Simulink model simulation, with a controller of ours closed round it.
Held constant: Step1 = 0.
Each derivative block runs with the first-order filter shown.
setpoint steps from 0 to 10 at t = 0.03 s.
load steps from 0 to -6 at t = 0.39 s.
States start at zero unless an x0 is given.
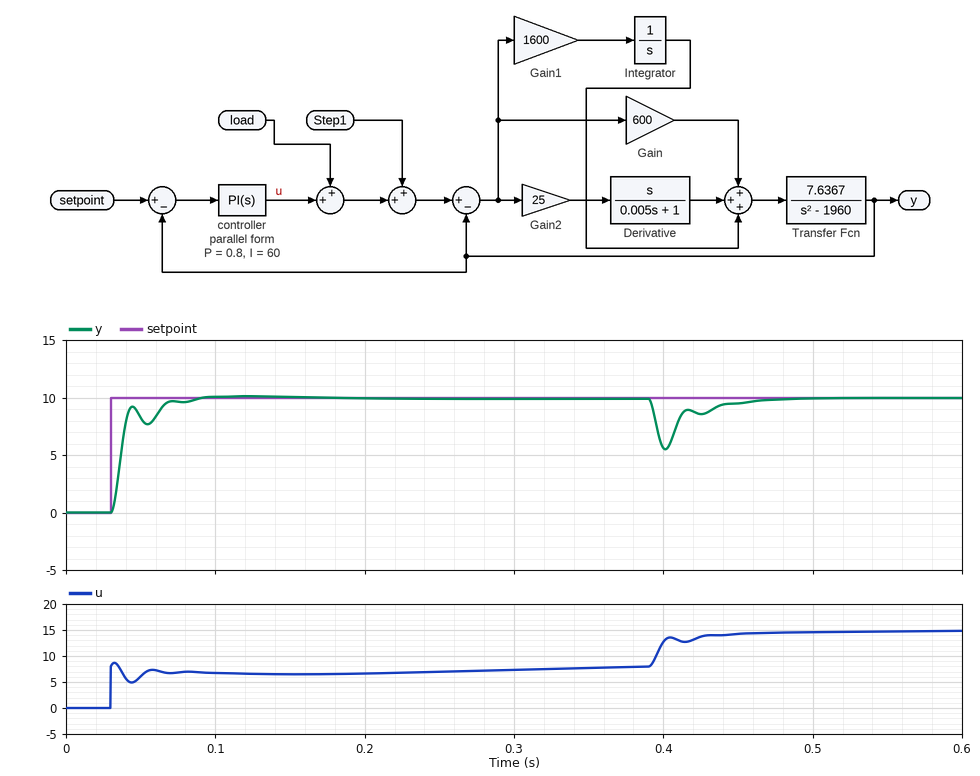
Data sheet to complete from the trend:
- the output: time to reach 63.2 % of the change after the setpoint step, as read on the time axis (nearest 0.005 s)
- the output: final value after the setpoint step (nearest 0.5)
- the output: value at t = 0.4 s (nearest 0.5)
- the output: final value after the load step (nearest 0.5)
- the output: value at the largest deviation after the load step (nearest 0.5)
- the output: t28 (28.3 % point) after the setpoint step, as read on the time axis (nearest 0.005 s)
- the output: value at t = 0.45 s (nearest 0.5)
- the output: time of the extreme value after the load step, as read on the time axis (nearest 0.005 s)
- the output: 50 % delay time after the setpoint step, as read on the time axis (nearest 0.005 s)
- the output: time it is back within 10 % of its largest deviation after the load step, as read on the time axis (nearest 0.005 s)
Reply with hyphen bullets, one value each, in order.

- 0.040 s
- 10.0
- 5.5
- 10.0
- 5.5
- 0.035 s
- 9.5
- 0.400 s
- 0.035 s
- 0.455 s
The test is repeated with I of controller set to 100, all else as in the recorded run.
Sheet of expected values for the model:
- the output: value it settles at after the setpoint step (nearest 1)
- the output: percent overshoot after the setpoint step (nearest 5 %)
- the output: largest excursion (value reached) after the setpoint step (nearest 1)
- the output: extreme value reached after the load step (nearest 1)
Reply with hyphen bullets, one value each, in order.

- 10
- 10 %
- 11
- 6
